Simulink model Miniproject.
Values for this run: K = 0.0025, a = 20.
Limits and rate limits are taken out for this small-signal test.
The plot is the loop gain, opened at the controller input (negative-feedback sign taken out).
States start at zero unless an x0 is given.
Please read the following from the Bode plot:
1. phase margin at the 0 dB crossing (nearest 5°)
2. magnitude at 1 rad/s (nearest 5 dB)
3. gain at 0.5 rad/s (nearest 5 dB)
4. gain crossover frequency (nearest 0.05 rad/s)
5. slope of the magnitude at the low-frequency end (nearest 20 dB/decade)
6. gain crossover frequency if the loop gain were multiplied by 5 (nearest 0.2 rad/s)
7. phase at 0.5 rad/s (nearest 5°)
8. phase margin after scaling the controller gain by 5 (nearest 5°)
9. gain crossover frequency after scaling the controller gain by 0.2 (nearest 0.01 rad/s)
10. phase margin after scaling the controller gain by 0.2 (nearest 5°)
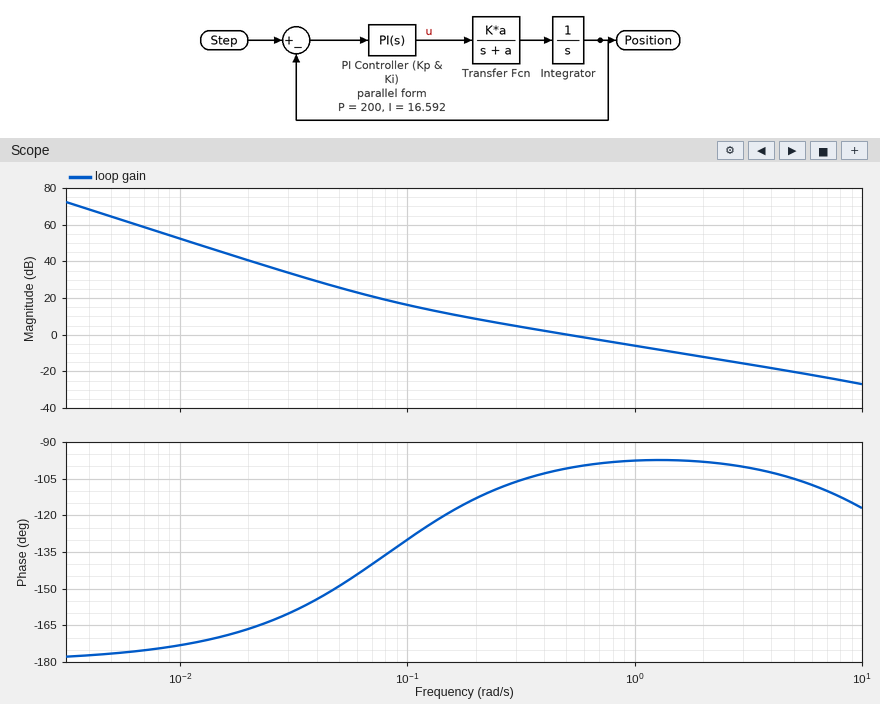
80°
-5 dB
0 dB
0.50 rad/s
-40 dB/decade
2.4 rad/s
-100°
80°
0.12 rad/s
55°
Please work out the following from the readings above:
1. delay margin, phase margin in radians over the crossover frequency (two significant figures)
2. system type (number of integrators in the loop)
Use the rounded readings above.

2.8 s
2
